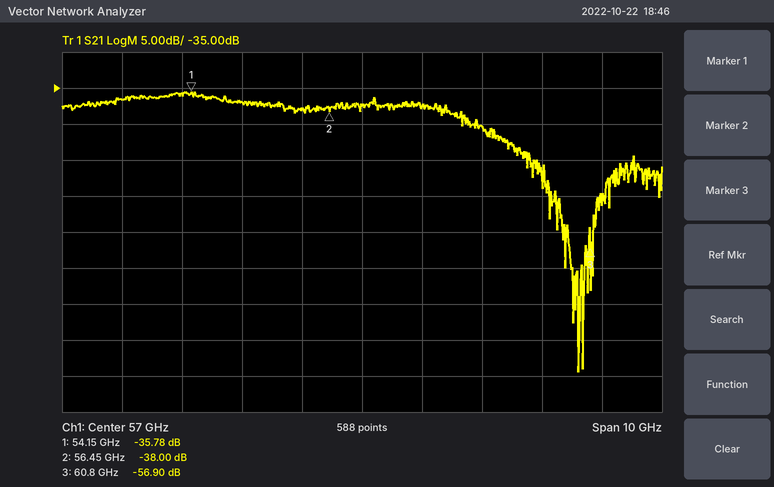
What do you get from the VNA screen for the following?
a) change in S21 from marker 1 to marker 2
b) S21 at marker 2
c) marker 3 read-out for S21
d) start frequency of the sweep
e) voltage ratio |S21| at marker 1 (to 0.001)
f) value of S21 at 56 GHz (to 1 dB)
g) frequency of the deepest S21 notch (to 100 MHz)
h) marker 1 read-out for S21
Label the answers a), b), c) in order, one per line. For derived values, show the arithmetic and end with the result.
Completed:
a) -38 − (-35.78) = -2.22 dB
b) -38.00 dB
c) -56.90 dB
d) 52 GHz
e) 10^(-35.78/20) ≈ 0.016
f) -38 dB
g) 60.6 GHz
h) -35.78 dB
